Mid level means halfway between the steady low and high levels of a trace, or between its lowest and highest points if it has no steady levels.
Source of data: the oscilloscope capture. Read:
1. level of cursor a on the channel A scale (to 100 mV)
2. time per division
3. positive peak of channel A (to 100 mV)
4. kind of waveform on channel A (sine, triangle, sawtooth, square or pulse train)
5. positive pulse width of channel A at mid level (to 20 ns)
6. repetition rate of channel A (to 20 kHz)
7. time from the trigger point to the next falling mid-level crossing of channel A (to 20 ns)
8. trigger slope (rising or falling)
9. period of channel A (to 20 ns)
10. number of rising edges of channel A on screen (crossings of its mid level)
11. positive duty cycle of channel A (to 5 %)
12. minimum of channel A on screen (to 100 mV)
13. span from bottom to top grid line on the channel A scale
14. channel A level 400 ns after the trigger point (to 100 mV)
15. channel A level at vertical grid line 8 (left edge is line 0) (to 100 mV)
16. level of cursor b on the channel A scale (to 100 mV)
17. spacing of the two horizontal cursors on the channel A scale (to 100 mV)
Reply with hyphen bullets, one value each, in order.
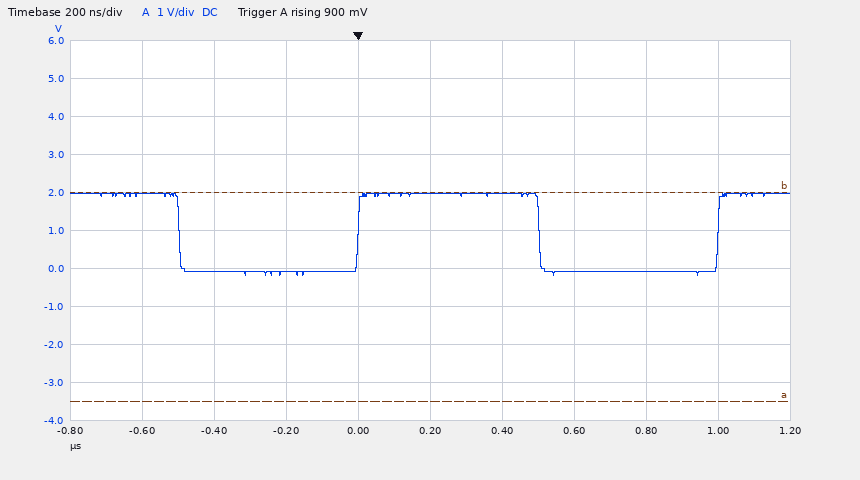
- -3.5 V
- 200 ns
- 2.0 V
- square
- 500 ns
- 1.00 MHz
- 500 ns
- rising
- 1.00 µs
- 2
- 50 %
- -200 mV
- 10 V
- 2.0 V
- -100 mV
- 2.0 V
- 5.5 V
